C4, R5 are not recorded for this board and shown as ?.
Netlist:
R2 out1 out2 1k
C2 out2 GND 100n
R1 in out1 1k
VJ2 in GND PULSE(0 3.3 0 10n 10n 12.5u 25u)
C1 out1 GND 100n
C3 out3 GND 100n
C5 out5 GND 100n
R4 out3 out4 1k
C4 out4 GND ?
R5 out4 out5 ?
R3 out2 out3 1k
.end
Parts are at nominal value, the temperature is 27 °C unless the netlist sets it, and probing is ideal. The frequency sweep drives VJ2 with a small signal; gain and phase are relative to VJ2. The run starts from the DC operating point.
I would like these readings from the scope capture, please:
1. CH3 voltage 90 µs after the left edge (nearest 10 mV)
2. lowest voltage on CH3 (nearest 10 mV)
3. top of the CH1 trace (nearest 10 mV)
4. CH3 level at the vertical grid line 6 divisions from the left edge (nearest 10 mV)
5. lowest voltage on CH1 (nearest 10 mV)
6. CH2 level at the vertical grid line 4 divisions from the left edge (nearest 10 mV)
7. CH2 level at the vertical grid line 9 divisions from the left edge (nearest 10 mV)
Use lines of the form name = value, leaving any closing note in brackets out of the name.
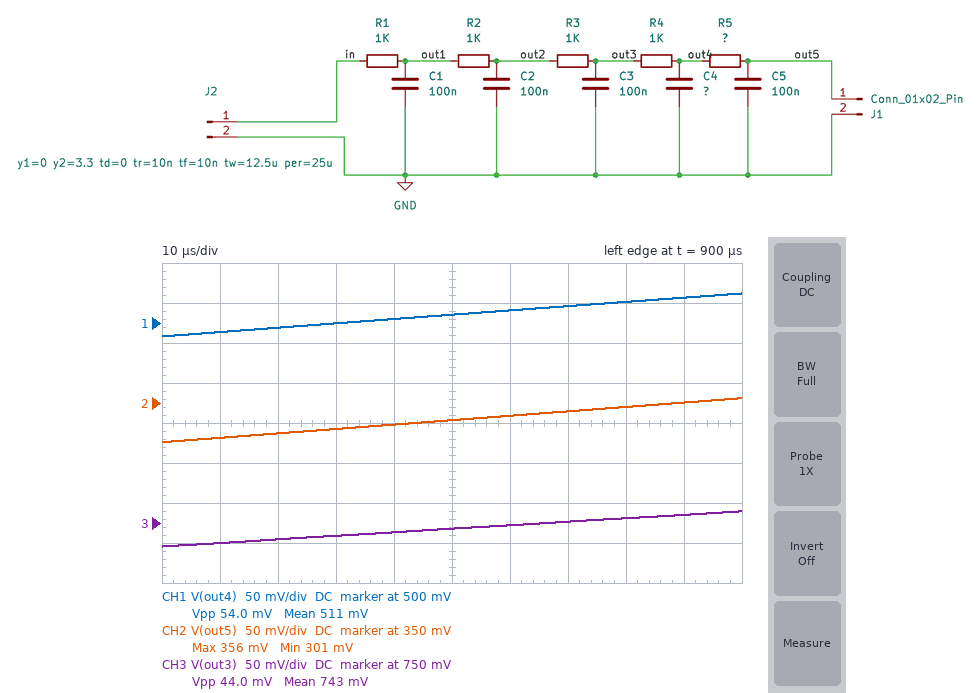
CH3 voltage 90 µs after the left edge = 760 mV
lowest voltage on CH3 = 720 mV
top of the CH1 trace = 540 mV
CH3 level at the vertical grid line 6 divisions from the left edge = 750 mV
lowest voltage on CH1 = 480 mV
CH2 level at the vertical grid line 4 divisions from the left edge = 320 mV
CH2 level at the vertical grid line 9 divisions from the left edge = 350 mV
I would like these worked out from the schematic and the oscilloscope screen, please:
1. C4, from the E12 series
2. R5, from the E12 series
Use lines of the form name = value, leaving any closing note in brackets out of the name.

C4, from the E12 series = 330 nF
R5, from the E12 series = 3.3 kΩ
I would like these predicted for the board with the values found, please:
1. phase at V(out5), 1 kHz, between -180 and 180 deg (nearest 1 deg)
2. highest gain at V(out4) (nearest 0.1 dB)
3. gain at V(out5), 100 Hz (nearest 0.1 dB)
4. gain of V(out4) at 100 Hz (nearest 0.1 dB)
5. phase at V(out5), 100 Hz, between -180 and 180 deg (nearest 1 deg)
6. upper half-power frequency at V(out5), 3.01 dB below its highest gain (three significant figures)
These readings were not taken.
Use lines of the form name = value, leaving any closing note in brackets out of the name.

phase at V(out5), 1 kHz, between -180 and 180 deg = 148 deg
highest gain at V(out4) = 0 dB
gain at V(out5), 100 Hz = -4.7 dB
gain of V(out4) at 100 Hz = -4.5 dB
phase at V(out5), 100 Hz, between -180 and 180 deg = -71 deg
upper half-power frequency at V(out5), 3.01 dB below its highest gain = 72.0 Hz
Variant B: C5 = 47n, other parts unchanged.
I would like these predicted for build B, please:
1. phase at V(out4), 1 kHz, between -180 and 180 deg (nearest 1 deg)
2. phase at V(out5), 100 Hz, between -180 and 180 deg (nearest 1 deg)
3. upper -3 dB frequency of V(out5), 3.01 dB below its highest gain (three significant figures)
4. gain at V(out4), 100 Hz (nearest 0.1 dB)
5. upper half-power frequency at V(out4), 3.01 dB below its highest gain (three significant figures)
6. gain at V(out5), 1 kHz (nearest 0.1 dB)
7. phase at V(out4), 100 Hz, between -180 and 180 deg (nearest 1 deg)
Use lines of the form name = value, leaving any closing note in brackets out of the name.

phase at V(out4), 1 kHz, between -180 and 180 deg = -150 deg
phase at V(out5), 100 Hz, between -180 and 180 deg = -63 deg
upper -3 dB frequency of V(out5), 3.01 dB below its highest gain = 82.6 Hz
gain at V(out4), 100 Hz = -3.9 dB
upper half-power frequency at V(out4), 3.01 dB below its highest gain = 83.1 Hz
gain at V(out5), 1 kHz = -27.1 dB
phase at V(out4), 100 Hz, between -180 and 180 deg = -57 deg
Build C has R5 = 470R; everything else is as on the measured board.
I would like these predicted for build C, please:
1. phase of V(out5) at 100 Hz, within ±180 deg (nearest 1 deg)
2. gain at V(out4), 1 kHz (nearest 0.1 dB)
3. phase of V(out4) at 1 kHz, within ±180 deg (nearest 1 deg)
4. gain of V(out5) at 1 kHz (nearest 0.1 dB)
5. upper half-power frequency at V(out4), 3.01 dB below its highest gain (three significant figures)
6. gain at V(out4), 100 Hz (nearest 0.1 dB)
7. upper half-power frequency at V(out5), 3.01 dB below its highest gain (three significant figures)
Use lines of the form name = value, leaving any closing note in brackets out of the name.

phase of V(out5) at 100 Hz, within ±180 deg = -62 deg
gain at V(out4), 1 kHz = -25.5 dB
phase of V(out4) at 1 kHz, within ±180 deg = -152 deg
gain of V(out5) at 1 kHz = -25.9 dB
upper half-power frequency at V(out4), 3.01 dB below its highest gain = 75.2 Hz
gain at V(out4), 100 Hz = -4.4 dB
upper half-power frequency at V(out5), 3.01 dB below its highest gain = 75.1 Hz
